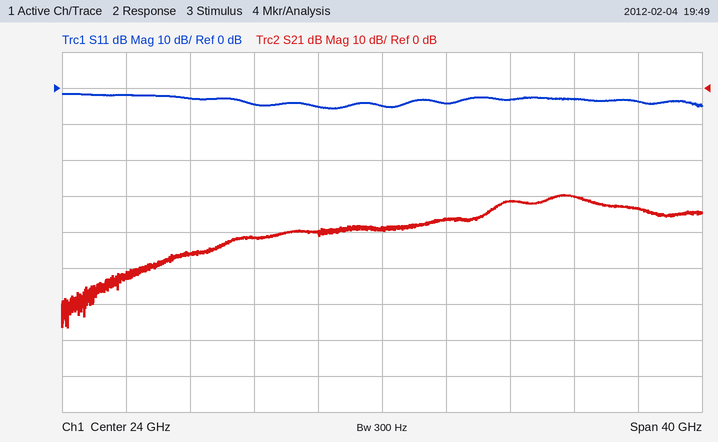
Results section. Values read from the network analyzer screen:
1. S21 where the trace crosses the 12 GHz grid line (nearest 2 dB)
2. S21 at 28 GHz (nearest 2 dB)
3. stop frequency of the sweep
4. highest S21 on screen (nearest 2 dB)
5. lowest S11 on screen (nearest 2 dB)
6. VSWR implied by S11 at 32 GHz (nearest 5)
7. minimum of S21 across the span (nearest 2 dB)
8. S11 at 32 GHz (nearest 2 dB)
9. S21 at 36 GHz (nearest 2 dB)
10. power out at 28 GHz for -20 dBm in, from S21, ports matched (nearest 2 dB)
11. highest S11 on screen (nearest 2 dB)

-46 dB
-36 dB
44 GHz
-30 dB
-6 dB
5
-66 dB
-4 dB
-30 dB
-56 dBm
-2 dB
